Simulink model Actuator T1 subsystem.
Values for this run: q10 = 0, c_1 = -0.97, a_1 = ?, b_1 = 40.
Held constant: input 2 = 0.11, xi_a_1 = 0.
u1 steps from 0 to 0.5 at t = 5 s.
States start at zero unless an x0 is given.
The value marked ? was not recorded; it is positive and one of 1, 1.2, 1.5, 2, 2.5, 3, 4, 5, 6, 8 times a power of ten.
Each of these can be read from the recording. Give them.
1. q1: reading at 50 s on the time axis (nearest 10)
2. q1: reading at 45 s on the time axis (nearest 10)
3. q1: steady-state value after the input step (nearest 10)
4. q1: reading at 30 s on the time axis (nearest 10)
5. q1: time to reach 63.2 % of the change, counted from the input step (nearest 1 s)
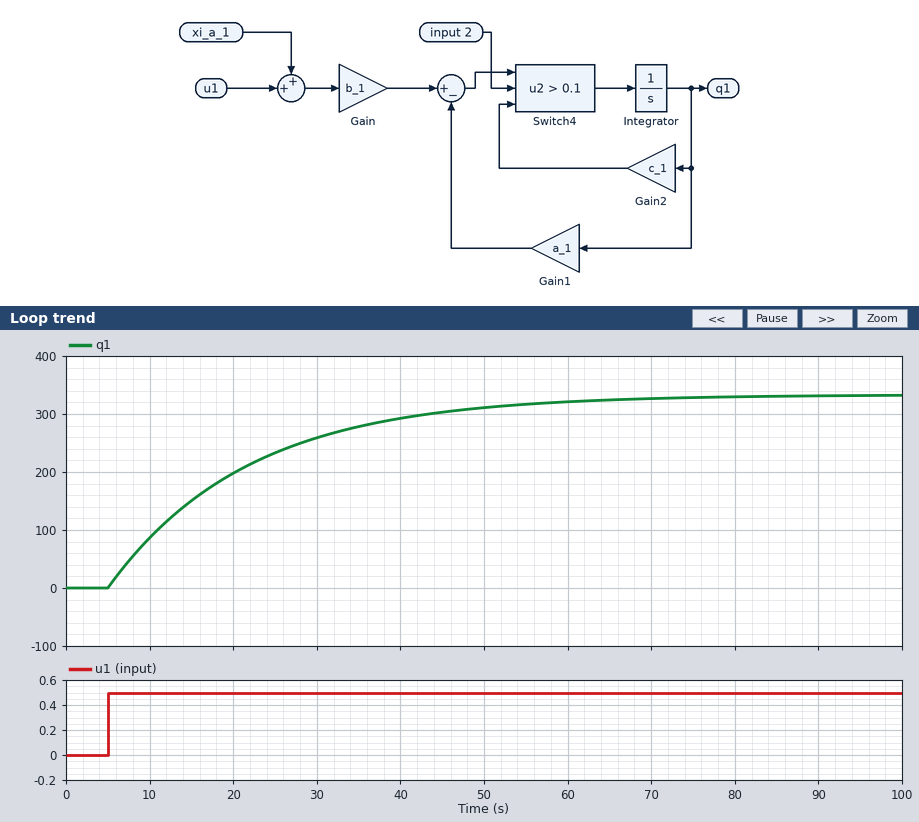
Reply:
310
300
330
260
17 s
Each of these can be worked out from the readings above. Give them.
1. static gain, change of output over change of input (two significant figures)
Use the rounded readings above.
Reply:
660
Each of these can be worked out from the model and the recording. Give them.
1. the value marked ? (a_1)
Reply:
0.06
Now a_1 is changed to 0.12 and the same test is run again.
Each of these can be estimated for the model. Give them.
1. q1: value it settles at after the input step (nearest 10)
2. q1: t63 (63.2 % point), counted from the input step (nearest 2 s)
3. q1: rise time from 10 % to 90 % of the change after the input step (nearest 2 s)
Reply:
170
8 s
18 s
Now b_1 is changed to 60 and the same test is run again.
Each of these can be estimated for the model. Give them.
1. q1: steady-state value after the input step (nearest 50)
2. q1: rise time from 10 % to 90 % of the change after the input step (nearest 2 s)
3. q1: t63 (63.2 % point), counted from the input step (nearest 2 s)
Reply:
500
36 s
16 s
